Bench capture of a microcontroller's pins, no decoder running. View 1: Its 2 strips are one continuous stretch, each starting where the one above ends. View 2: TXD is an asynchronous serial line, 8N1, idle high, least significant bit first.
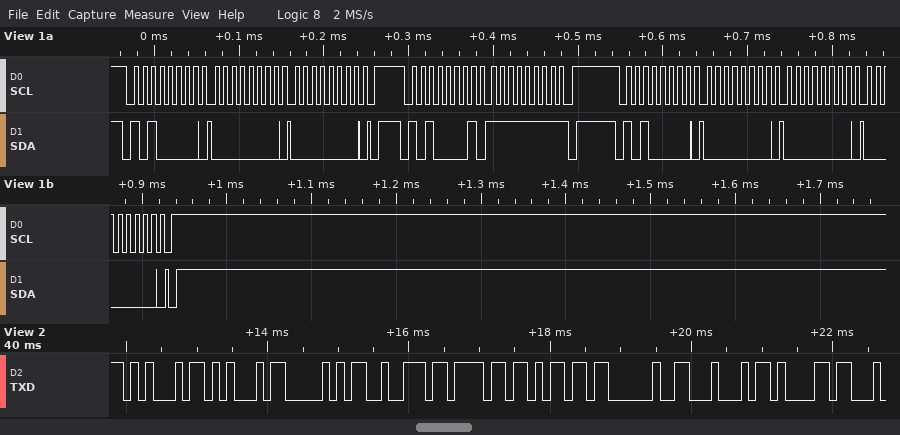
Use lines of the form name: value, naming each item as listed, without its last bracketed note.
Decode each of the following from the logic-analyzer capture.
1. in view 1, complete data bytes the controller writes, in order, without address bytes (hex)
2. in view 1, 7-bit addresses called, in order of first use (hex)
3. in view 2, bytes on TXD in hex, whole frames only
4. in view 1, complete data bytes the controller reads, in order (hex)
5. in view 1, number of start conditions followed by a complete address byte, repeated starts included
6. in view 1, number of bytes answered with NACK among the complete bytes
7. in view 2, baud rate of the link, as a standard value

in view 1, complete data bytes the controller writes, in order, without address bytes: 00 00 00 00 00
in view 1, 7-bit addresses called, in order of first use: 0x50
in view 2, bytes on TXD in hex, whole frames only: 45 45 50 72 6F 6D 20 44 61
in view 1, complete data bytes the controller reads, in order: FF
in view 1, number of start conditions followed by a complete address byte, repeated starts included: 3
in view 1, number of bytes answered with NACK among the complete bytes: 1
in view 2, baud rate of the link, as a standard value: 9600 baud
